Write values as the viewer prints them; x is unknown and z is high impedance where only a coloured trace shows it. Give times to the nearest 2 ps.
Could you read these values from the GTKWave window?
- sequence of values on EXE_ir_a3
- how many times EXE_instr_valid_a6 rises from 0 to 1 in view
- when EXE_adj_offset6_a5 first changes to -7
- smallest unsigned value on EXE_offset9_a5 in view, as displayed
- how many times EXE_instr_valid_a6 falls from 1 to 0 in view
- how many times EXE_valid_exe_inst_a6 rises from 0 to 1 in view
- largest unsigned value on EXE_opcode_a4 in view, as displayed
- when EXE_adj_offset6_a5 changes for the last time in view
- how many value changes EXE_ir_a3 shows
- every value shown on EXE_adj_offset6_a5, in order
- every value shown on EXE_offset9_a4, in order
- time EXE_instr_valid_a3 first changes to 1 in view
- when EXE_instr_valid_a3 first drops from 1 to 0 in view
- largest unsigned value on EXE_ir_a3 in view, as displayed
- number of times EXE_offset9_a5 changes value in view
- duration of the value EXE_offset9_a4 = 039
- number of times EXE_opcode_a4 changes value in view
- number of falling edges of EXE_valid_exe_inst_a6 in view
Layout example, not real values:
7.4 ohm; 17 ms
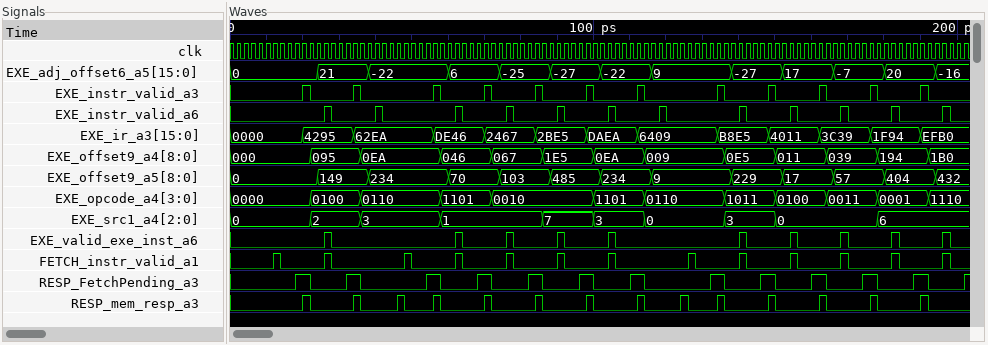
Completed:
0000, 4295, 62EA, DE46, 2467, 2BE5, DAEA, 6409, B8E5, 4011, 3C39, 1F94, EFB0; 12; 166 ps; 0; 12; 10; 1110; 194 ps; 12; 0, 21, -22, 6, -25, -27, -22, 9, -27, 17, -7, 20, -16; 000, 095, 0EA, 046, 067, 1E5, 0EA, 009, 0E5, 011, 039, 194, 1B0; 20 ps; 22 ps; EFB0; 12; 14 ps; 11; 10
